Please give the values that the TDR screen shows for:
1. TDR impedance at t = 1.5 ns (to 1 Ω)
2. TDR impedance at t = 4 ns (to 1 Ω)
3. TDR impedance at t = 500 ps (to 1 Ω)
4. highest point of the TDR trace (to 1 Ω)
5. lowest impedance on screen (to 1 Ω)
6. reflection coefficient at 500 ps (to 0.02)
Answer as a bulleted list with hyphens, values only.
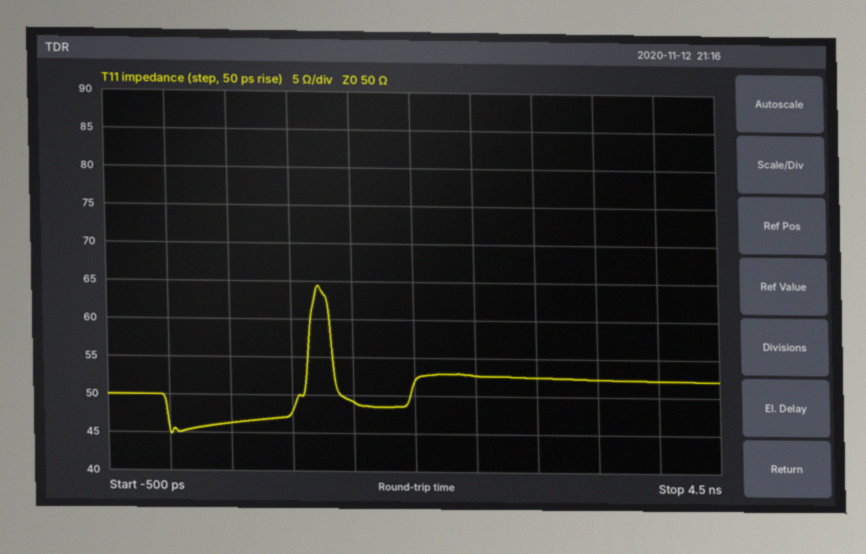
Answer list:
- 49 Ω
- 52 Ω
- 46 Ω
- 64 Ω
- 45 Ω
- -0.04
